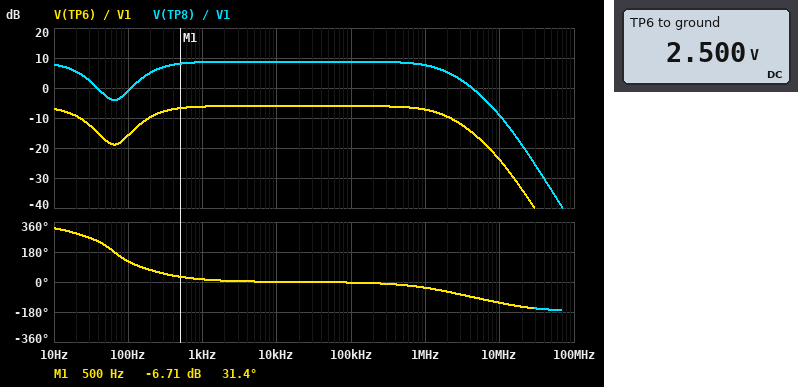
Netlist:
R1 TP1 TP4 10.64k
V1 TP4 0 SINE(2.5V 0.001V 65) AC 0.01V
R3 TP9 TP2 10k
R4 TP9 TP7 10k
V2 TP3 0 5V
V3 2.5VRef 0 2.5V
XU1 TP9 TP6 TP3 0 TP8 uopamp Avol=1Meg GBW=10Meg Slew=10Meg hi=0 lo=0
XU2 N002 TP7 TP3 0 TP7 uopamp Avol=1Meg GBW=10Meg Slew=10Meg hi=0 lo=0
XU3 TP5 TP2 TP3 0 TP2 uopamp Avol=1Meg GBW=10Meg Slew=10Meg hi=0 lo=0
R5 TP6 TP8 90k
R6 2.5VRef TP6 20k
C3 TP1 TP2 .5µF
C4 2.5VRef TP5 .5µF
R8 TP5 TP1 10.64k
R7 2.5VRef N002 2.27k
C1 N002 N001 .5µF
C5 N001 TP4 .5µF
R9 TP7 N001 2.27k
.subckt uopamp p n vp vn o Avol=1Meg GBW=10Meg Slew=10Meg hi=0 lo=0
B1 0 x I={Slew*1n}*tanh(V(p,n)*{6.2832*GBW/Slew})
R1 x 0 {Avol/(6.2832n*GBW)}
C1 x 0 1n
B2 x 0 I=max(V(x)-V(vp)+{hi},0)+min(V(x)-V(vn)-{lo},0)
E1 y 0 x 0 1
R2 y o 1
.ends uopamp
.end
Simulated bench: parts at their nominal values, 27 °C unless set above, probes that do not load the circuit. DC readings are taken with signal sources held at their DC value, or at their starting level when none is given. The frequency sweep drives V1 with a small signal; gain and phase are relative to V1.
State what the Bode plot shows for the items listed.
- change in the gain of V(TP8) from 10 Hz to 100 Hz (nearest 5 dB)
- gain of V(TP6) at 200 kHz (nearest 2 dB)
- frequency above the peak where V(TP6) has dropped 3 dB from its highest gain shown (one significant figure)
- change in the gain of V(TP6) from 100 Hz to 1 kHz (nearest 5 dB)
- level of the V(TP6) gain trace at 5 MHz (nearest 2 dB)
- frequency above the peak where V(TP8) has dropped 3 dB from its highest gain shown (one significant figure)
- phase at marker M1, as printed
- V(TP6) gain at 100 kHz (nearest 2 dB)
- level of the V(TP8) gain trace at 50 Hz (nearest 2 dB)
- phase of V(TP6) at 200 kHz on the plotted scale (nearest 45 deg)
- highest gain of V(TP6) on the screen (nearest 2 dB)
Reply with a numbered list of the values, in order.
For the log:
1. -10 dB
2. -6 dB
3. 2 MHz
4. 10 dB
5. -16 dB
6. 2 MHz
7. 31.4 deg
8. -6 dB
9. -2 dB
10. 0 deg
11. -6 dB
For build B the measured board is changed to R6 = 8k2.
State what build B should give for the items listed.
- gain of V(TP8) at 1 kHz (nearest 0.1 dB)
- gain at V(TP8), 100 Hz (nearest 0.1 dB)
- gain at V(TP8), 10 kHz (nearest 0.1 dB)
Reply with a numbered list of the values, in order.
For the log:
1. 15.4 dB
2. 5.8 dB
3. 15.5 dB
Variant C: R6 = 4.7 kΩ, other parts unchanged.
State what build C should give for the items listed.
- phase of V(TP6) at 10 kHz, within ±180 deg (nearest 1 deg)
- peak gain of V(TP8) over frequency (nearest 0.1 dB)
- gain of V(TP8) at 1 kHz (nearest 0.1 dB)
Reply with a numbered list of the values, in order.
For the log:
1. 0 deg
2. 20.1 dB
3. 19.9 dB
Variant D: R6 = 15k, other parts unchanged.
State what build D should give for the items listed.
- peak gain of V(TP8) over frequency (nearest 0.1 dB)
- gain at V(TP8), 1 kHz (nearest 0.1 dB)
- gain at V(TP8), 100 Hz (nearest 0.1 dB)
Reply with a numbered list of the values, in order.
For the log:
1. 10.9 dB
2. 10.7 dB
3. 1.2 dB
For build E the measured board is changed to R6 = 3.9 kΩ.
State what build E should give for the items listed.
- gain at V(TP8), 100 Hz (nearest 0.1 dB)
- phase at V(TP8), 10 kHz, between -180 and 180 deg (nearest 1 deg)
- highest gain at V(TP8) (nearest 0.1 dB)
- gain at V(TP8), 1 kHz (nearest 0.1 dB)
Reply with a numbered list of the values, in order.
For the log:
1. 11.9 dB
2. 0 deg
3. 21.6 dB
4. 21.4 dB
